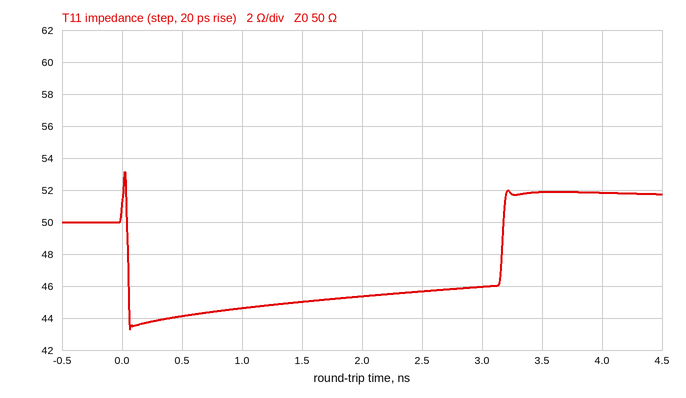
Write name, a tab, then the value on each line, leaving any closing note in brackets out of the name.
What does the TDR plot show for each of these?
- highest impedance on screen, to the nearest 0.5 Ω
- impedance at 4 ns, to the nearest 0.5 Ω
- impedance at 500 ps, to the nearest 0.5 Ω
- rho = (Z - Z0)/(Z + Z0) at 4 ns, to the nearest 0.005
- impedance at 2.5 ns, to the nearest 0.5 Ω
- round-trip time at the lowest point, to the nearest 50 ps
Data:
highest impedance on screen, to the nearest 0.5 Ω	53.0 Ω
impedance at 4 ns, to the nearest 0.5 Ω	52.0 Ω
impedance at 500 ps, to the nearest 0.5 Ω	44.0 Ω
rho = (Z - Z0)/(Z + Z0) at 4 ns, to the nearest 0.005	+0.020
impedance at 2.5 ns, to the nearest 0.5 Ω	45.5 Ω
round-trip time at the lowest point, to the nearest 50 ps	50 ps
